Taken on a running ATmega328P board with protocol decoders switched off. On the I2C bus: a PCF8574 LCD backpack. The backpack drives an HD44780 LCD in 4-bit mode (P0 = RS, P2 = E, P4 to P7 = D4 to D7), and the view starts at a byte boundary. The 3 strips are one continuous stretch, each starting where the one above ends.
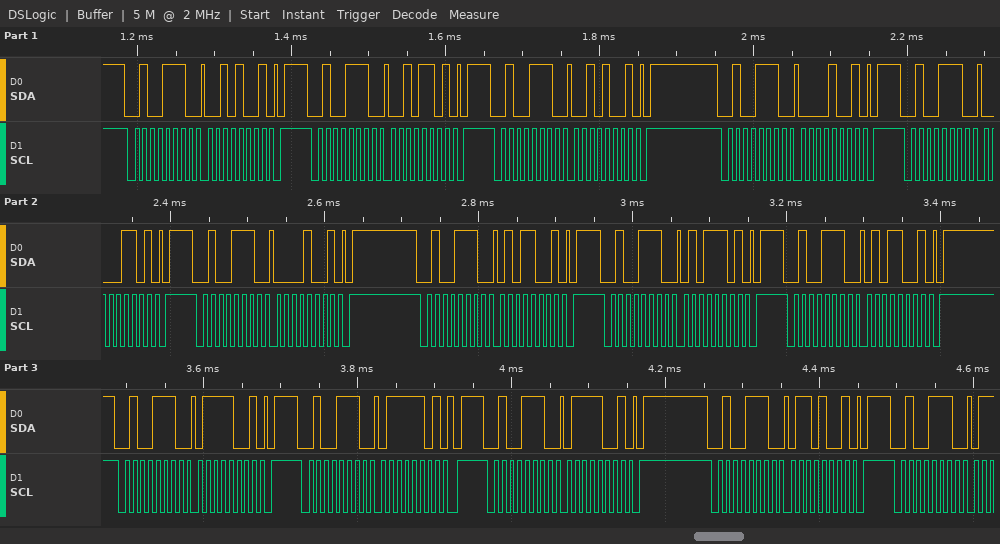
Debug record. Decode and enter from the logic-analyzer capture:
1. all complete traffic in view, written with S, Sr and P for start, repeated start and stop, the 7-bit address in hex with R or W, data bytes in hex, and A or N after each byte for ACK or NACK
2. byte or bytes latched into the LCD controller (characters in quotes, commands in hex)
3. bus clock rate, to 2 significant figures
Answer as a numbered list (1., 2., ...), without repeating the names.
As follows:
1. S 27W A 29 A P S 27W A 2D A P S 27W A 29 A P S 27W A 09 A P S 27W A 0D A P S 27W A 09 A P S 27W A 59 A P S 27W A 5D A P S 27W A 59 A P S 27W A 79 A P S 27W A 7D A P S 27W A 79 A P S 27W A 69 A P S 27W A
2. ' ' 'W'
3. 100 kHz
